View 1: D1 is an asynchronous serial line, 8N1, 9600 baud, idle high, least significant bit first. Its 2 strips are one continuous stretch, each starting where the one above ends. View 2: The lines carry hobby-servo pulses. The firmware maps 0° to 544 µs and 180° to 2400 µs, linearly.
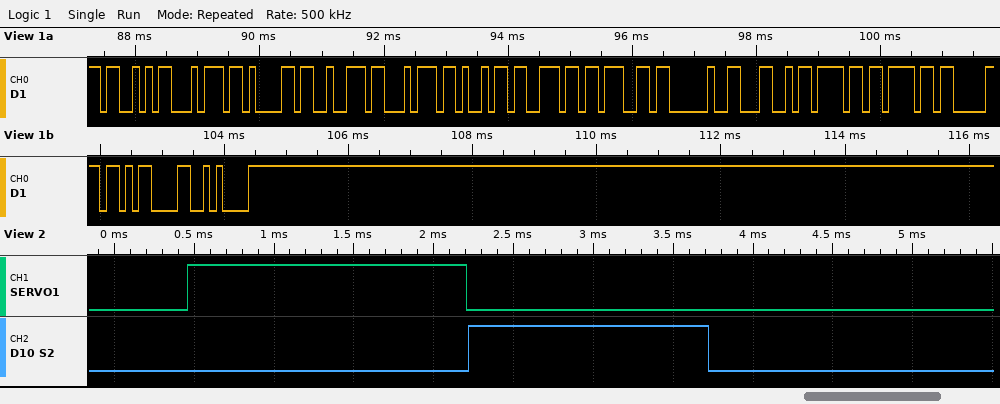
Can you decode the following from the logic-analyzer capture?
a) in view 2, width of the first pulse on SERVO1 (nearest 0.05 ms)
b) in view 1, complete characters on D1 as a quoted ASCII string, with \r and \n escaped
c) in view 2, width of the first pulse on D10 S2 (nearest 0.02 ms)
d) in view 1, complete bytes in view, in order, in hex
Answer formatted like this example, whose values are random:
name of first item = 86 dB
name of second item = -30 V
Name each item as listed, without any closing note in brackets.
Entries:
in view 2, width of the first pulse on SERVO1 = 1.75 ms
in view 1, complete characters on D1 as a quoted ASCII string, with \r and \n escaped = "Starting Loop\r\n"
in view 2, width of the first pulse on D10 S2 = 1.50 ms
in view 1, complete bytes in view, in order, in hex = 53 74 61 72 74 69 6E 67 20 4C 6F 6F 70 0D 0A
